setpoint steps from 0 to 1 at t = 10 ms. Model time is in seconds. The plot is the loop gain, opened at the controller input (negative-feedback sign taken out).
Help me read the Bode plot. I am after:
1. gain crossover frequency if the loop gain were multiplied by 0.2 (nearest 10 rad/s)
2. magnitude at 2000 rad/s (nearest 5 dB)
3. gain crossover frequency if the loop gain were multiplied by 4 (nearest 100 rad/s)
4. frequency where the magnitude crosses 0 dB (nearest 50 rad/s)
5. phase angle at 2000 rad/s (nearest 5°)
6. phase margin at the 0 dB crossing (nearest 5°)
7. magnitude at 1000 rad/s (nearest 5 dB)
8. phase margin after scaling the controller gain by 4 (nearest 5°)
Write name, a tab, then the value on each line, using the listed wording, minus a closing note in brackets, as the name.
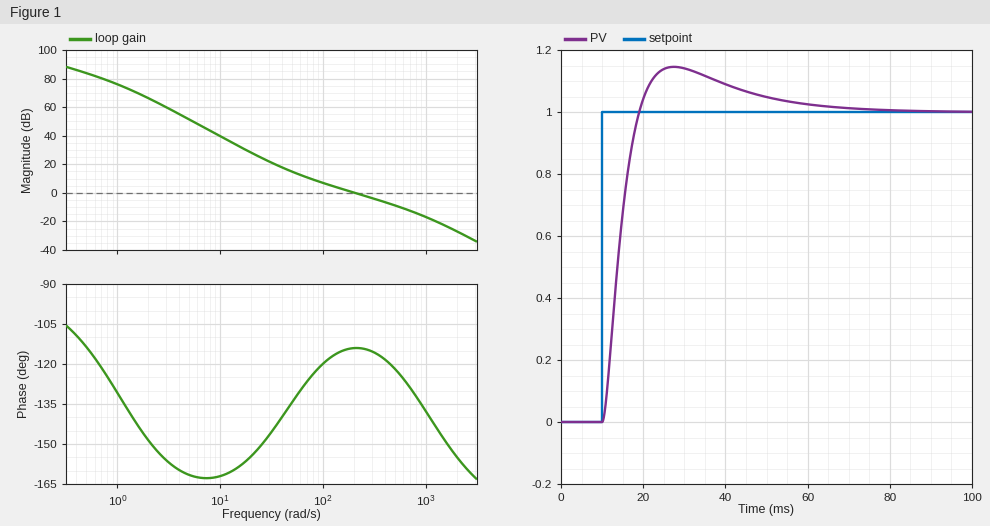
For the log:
gain crossover frequency if the loop gain were multiplied by 0.2	50 rad/s
magnitude at 2000 rad/s	-25 dB
gain crossover frequency if the loop gain were multiplied by 4	700 rad/s
frequency where the magnitude crosses 0 dB	200 rad/s
phase angle at 2000 rad/s	-155°
phase margin at the 0 dB crossing	65°
magnitude at 1000 rad/s	-15 dB
phase margin after scaling the controller gain by 4	50°
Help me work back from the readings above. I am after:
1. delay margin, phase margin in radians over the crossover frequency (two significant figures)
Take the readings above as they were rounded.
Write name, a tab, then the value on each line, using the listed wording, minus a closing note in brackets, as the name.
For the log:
delay margin, phase margin in radians over the crossover frequency	0.0057 s
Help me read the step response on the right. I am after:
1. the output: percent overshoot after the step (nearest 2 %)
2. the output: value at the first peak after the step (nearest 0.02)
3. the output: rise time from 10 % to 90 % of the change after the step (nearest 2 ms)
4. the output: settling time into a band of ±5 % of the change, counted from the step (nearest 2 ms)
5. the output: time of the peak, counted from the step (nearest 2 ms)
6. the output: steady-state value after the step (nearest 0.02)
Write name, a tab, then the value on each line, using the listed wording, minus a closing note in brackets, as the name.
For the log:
the output: percent overshoot after the step	14 %
the output: value at the first peak after the step	1.14
the output: rise time from 10 % to 90 % of the change after the step	6 ms
the output: settling time into a band of ±5 % of the change, counted from the step	40 ms
the output: time of the peak, counted from the step	18 ms
the output: steady-state value after the step	1.00
